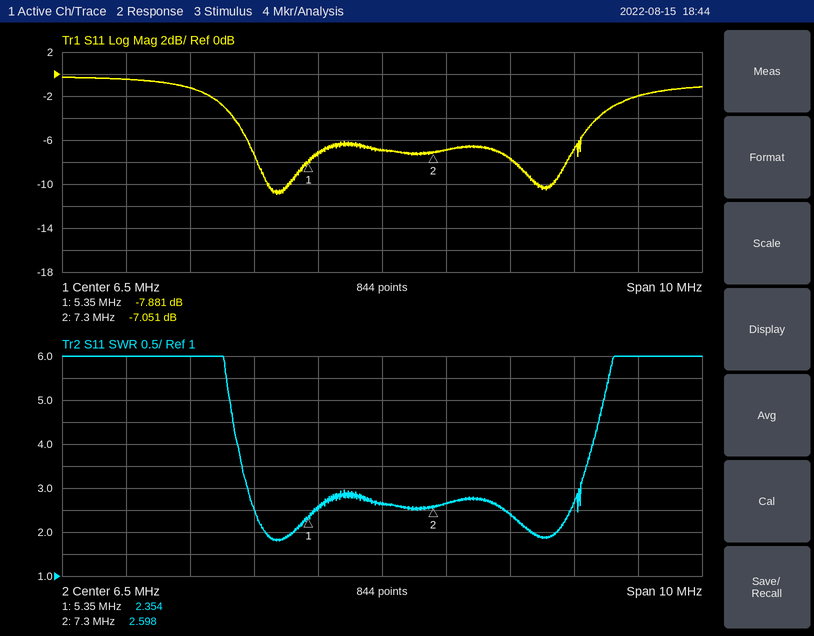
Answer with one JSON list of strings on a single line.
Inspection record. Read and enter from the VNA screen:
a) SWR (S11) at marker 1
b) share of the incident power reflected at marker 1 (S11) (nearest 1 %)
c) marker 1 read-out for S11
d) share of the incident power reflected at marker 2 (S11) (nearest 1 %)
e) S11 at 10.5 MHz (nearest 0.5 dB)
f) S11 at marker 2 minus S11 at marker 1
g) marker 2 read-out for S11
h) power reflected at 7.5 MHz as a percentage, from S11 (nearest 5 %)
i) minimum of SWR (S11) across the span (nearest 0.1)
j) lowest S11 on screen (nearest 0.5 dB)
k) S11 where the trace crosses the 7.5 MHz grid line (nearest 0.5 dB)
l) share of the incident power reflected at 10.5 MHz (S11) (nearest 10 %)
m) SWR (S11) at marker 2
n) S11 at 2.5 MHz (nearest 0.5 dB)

["2.354", "16 %", "-7.881 dB", "20 %", "-2.0 dB", "0.830 dB", "-7.051 dB", "20 %", "1.8", "-11.0 dB", "-7.0 dB", "60 %", "2.598", "-0.5 dB"]
